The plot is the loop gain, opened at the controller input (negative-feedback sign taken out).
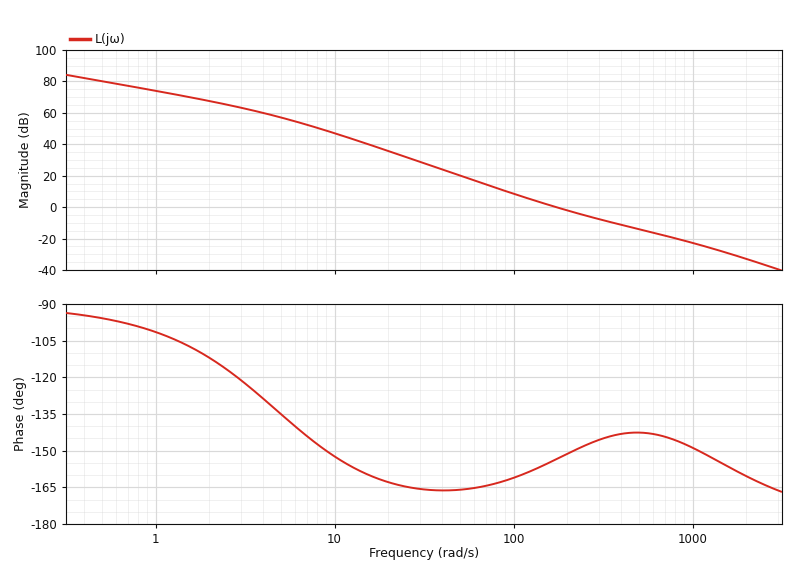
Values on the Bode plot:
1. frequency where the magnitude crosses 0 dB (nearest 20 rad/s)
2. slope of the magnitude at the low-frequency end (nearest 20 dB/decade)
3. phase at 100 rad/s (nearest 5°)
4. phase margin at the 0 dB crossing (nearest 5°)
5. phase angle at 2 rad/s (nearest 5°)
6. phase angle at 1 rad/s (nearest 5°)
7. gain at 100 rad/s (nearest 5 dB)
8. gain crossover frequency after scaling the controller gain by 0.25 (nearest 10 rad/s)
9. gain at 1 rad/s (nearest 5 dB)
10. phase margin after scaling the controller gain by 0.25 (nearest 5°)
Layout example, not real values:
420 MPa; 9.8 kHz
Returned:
180 rad/s; -20 dB/decade; -160°; 25°; -110°; -100°; 10 dB; 80 rad/s; 75 dB; 15°
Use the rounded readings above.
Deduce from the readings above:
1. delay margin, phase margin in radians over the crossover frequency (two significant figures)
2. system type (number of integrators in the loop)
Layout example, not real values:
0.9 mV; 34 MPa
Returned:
0.0024 s; 1
